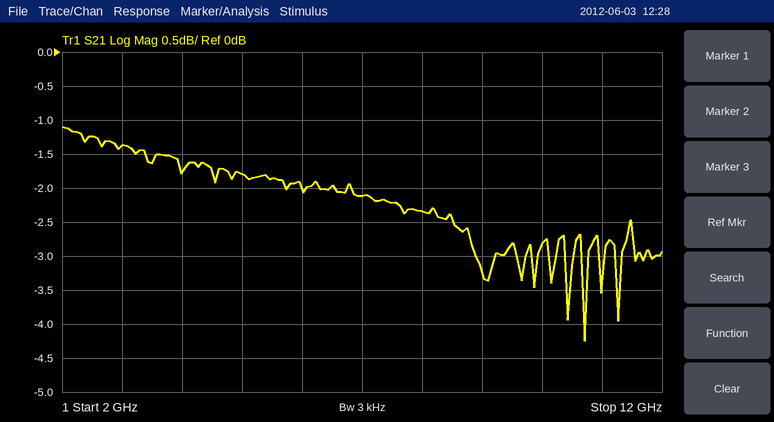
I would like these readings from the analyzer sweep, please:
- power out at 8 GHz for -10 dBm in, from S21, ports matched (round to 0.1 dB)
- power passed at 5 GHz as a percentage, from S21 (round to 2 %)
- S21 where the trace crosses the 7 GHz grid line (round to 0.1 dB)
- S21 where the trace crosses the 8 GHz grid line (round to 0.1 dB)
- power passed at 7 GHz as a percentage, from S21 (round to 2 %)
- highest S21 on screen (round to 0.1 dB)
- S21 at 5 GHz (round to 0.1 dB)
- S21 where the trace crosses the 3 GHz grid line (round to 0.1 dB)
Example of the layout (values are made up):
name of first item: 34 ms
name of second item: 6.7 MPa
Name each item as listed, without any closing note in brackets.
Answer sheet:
power out at 8 GHz for -10 dBm in, from S21, ports matched: -12.3 dBm
power passed at 5 GHz as a percentage, from S21: 66 %
S21 where the trace crosses the 7 GHz grid line: -2.1 dB
S21 where the trace crosses the 8 GHz grid line: -2.3 dB
power passed at 7 GHz as a percentage, from S21: 62 %
highest S21 on screen: -1.1 dB
S21 at 5 GHz: -1.8 dB
S21 where the trace crosses the 3 GHz grid line: -1.4 dB
